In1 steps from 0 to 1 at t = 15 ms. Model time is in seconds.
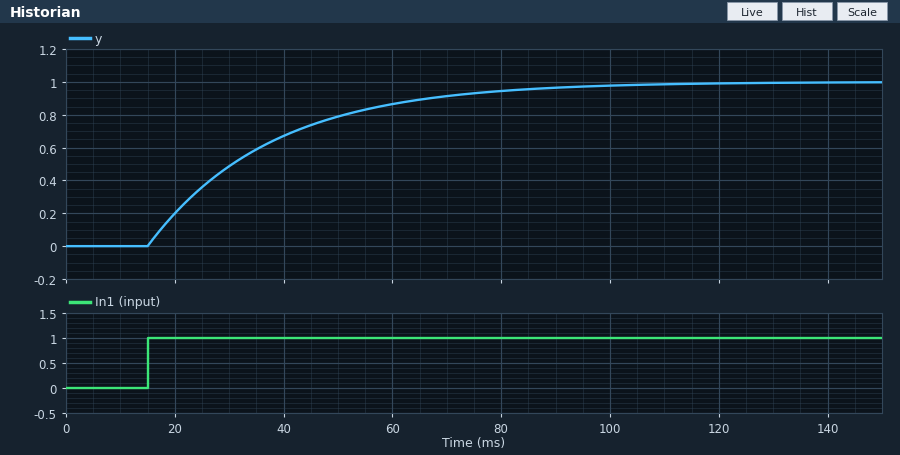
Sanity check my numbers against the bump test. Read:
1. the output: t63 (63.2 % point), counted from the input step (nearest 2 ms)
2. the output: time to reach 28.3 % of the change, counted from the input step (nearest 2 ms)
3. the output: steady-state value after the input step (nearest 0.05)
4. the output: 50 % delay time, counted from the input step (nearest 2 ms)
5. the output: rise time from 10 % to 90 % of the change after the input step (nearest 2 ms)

22 ms
8 ms
1.00
16 ms
50 ms
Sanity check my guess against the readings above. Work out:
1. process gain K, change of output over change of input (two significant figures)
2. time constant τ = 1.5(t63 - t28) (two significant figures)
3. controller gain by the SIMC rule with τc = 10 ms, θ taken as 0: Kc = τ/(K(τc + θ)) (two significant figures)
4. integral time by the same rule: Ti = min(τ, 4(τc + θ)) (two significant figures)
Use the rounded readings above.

1.0
21 ms
2.1
21 ms
